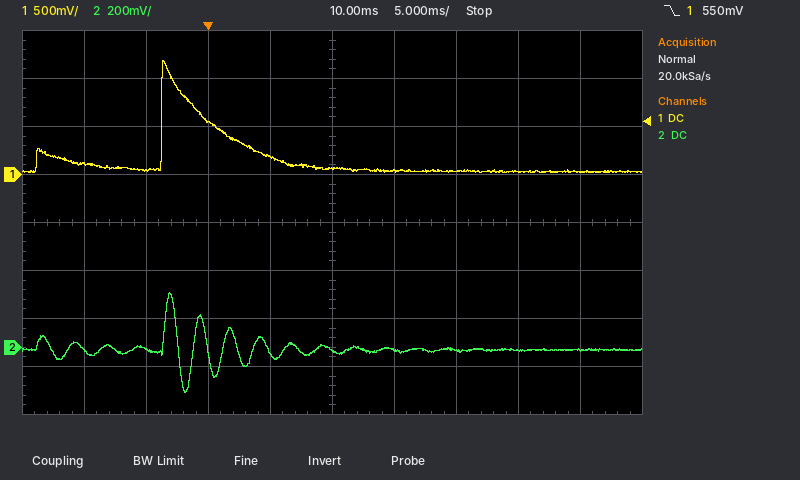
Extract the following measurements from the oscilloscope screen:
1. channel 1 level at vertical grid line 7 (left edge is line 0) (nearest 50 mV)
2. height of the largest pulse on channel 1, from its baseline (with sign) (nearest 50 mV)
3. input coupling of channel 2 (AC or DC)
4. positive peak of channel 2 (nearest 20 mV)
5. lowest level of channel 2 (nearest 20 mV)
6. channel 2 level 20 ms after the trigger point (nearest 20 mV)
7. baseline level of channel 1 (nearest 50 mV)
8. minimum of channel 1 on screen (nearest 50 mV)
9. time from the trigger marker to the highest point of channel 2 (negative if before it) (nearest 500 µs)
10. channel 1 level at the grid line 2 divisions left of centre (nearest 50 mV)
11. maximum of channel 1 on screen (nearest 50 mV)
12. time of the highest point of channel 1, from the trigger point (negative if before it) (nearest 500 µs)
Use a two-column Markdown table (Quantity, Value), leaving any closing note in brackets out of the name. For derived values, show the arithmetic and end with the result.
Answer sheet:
| Quantity | Value |
|---|---|
| channel 1 level at vertical grid line 7 (left edge is line 0) | 50 mV |
| height of the largest pulse on channel 1, from its baseline (with sign) | 1.20 V − (50 mV) = +1.15 V |
| input coupling of channel 2 | DC |
| positive peak of channel 2 | 220 mV |
| lowest level of channel 2 | -180 mV |
| channel 2 level 20 ms after the trigger point | -20 mV |
| baseline level of channel 1 | 50 mV |
| minimum of channel 1 on screen | 0 mV |
| time from the trigger marker to the highest point of channel 2 (negative if before it) | -3.0 ms |
| channel 1 level at the grid line 2 divisions left of centre | 550 mV |
| maximum of channel 1 on screen | 1.20 V |
| time of the highest point of channel 1, from the trigger point (negative if before it) | -3.5 ms |
